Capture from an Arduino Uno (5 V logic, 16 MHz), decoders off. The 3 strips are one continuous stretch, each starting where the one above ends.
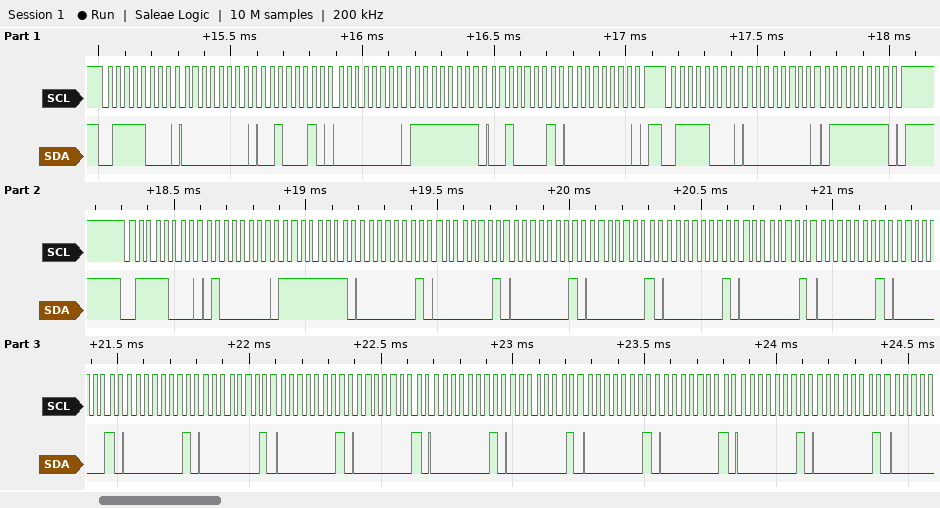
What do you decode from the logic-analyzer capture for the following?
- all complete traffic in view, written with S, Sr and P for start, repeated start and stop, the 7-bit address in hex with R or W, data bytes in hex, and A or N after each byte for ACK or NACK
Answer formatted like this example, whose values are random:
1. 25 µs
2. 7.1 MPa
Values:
1. S 3CW A 00 A 22 A 00 A FF A 21 A 00 A P S 3CW A 00 A 7F A P S 3CW A 40 A FF A 01 A 01 A 01 A 01 A 01 A 01 A 01 A 01 A 01 A 01 A 01 A 01 A 01 A 01 A 01 A 01 A 01 A 01 A
